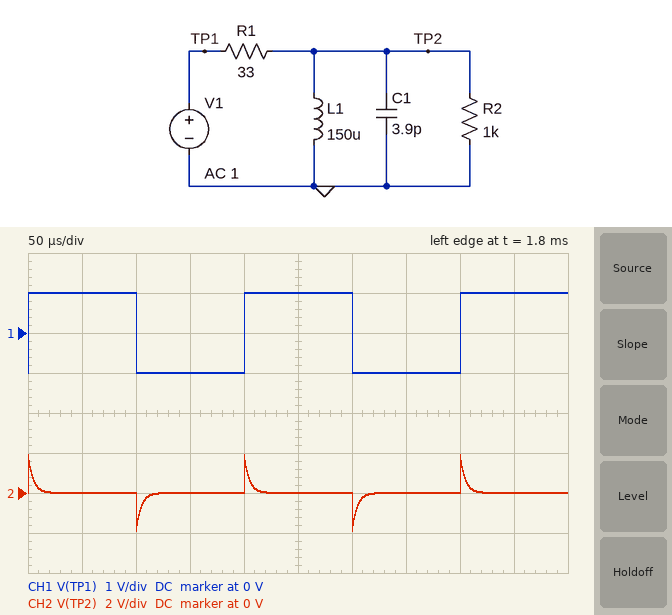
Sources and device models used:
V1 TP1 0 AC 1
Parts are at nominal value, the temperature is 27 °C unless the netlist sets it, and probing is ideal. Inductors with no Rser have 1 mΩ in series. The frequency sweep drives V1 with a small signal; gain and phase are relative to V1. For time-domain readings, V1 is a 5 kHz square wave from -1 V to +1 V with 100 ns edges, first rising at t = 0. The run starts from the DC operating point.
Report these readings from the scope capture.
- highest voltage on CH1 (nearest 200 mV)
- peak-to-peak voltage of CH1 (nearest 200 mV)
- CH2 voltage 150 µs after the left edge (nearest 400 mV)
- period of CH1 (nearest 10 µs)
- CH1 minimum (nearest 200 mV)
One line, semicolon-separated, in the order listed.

1.0 V; 2.0 V; 0 V; 200 µs; -1.0 V
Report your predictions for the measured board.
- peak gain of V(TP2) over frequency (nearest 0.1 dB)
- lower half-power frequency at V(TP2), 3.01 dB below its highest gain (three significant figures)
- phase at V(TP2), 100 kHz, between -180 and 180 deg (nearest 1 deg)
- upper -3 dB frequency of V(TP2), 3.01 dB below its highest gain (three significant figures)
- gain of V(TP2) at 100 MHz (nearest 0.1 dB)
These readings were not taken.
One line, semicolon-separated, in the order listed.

-0.3 dB; 33.9 kHz; 19 deg; 1.28 GHz; -0.3 dB
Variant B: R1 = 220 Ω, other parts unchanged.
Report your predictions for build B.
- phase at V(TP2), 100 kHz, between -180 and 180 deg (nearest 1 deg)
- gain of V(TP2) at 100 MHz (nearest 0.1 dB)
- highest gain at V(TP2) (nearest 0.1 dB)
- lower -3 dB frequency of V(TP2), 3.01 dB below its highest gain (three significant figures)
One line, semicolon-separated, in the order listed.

62 deg; -2.5 dB; -1.7 dB; 191 kHz
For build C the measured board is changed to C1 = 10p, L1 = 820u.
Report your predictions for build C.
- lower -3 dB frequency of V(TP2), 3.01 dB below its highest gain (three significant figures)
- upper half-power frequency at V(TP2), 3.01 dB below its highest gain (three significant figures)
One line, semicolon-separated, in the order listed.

6.20 kHz; 498 MHz
